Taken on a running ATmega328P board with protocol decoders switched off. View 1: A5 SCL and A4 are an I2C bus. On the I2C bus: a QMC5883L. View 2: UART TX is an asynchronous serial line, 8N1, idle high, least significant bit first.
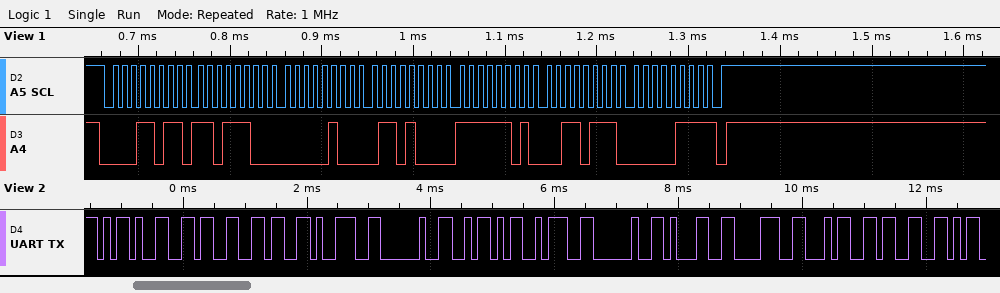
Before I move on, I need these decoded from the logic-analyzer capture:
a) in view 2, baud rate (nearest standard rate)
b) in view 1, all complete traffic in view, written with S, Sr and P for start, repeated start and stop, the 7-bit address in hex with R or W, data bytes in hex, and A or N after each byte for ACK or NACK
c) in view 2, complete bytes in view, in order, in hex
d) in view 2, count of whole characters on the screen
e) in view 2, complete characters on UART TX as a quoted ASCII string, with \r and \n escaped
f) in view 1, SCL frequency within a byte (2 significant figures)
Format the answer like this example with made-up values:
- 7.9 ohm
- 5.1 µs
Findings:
- 9600 baud
- S 0DR A DC A 04 A 68 A FD A 37 A 07 N P
- 2D 36 36 39 20 5A 3A 20 31 38 34 33
- 12
- "-669 Z: 1843"
- 100 kHz
